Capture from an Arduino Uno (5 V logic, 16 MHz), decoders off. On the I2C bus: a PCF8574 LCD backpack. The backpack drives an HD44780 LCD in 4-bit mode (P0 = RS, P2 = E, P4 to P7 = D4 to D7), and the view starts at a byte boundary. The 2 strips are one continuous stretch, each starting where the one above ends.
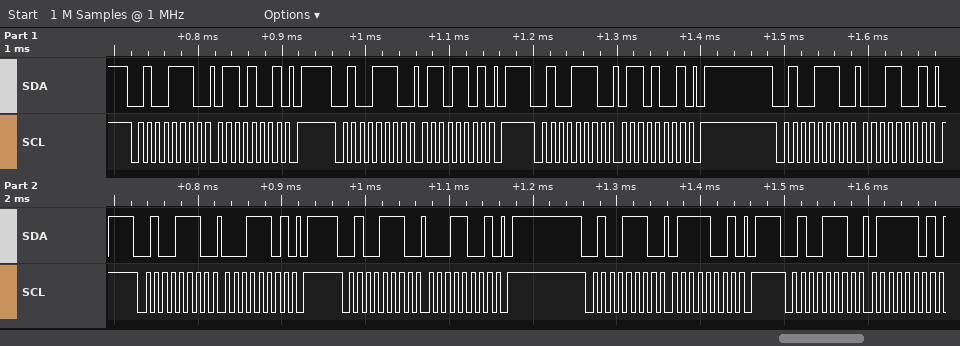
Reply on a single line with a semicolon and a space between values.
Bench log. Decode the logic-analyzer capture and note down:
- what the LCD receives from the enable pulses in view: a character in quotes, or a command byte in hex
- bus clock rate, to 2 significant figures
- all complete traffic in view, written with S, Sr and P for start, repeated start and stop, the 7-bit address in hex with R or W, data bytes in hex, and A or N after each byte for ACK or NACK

'a'; 100 kHz; S 27W A 69 A P S 27W A 6D A P S 27W A 69 A P S 27W A 19 A P S 27W A 1D A P S 27W A 19 A P S 27W A 79 A P S 27W A 7D A
